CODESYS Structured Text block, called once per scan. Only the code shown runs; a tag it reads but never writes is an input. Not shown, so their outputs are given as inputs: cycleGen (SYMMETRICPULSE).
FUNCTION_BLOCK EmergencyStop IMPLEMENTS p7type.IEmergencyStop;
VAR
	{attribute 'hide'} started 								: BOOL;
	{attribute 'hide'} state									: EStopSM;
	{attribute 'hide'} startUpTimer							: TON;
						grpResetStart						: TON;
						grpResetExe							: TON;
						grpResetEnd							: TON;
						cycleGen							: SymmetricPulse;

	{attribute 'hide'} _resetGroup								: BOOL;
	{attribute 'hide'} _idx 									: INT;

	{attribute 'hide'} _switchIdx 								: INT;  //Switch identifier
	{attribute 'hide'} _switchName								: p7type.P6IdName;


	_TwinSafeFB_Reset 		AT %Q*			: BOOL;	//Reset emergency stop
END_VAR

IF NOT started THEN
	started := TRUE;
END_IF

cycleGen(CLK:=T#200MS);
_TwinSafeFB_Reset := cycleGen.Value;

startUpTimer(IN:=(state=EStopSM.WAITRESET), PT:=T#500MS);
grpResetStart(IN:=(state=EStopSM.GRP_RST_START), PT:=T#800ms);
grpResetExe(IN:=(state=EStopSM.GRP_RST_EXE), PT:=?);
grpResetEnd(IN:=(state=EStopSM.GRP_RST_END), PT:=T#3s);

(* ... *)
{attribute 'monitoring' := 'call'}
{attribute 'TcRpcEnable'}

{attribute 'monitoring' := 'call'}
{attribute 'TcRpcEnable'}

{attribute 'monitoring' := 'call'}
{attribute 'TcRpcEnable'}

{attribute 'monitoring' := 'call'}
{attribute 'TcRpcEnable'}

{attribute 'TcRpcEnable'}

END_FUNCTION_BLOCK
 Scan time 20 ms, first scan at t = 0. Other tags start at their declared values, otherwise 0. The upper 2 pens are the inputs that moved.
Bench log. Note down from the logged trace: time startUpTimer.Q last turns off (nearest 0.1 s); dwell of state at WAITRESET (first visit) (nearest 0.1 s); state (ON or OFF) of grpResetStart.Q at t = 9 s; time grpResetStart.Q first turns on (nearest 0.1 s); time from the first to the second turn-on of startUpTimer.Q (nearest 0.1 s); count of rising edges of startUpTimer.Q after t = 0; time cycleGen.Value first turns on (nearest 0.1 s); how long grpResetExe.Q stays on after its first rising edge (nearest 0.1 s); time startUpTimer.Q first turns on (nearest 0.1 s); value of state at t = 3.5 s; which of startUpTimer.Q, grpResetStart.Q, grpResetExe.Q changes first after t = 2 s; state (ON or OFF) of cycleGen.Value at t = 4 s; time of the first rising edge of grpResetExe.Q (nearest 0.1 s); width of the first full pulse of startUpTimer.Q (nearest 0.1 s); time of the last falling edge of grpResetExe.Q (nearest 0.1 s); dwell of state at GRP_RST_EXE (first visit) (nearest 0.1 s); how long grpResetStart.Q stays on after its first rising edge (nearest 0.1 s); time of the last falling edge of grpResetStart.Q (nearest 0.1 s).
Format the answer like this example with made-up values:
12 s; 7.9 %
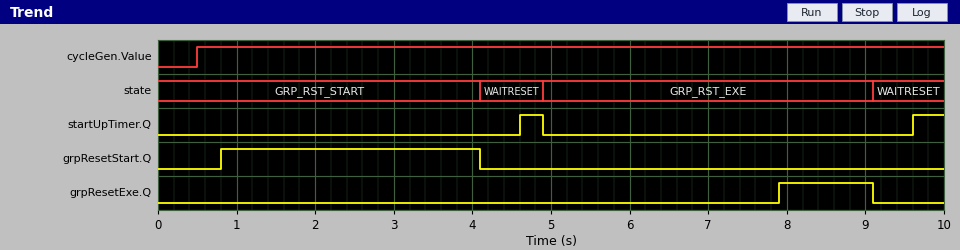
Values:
4.9 s; 0.8 s; OFF; 0.8 s; 5.0 s; 2; 0.5 s; 1.2 s; 4.6 s; GRP_RST_START; grpResetStart.Q; ON; 7.9 s; 0.3 s; 9.1 s; 4.2 s; 3.3 s; 4.1 s
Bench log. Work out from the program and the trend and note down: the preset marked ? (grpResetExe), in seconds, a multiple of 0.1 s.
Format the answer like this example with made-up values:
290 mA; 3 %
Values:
3.0 s
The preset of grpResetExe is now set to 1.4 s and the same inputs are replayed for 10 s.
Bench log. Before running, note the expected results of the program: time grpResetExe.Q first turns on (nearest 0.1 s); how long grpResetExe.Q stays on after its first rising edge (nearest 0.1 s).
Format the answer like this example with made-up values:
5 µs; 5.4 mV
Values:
6.3 s; 2.8 s
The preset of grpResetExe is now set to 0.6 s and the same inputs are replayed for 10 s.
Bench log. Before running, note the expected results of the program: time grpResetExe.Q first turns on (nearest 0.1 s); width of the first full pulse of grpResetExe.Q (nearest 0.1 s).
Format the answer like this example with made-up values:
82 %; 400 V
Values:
5.5 s; 3.6 s
